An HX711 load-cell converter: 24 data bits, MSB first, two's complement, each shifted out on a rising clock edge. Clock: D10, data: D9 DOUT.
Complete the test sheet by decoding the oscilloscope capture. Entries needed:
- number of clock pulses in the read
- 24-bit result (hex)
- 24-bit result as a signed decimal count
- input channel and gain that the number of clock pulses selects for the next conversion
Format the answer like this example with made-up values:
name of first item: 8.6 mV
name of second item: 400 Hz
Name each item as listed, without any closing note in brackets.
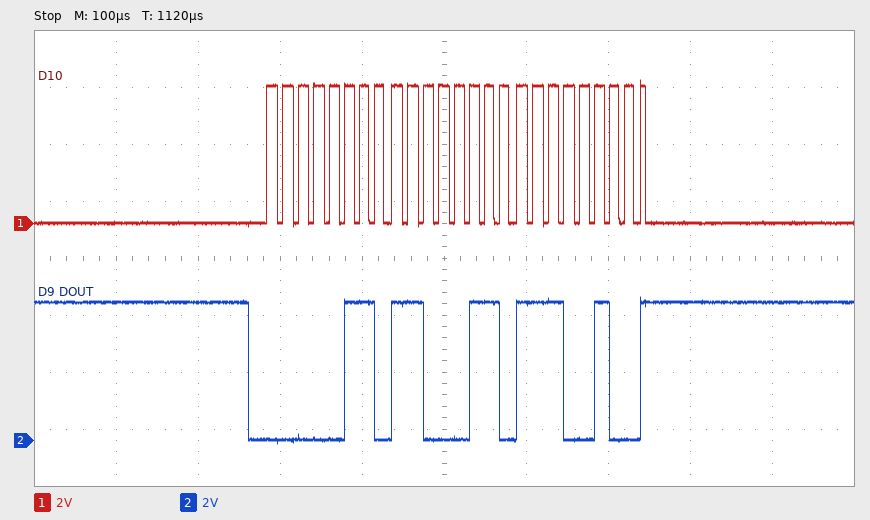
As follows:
number of clock pulses in the read: 25
24-bit result: 0x06C6E4
24-bit result as a signed decimal count: 444132
input channel and gain that the number of clock pulses selects for the next conversion: channel A, gain 128
